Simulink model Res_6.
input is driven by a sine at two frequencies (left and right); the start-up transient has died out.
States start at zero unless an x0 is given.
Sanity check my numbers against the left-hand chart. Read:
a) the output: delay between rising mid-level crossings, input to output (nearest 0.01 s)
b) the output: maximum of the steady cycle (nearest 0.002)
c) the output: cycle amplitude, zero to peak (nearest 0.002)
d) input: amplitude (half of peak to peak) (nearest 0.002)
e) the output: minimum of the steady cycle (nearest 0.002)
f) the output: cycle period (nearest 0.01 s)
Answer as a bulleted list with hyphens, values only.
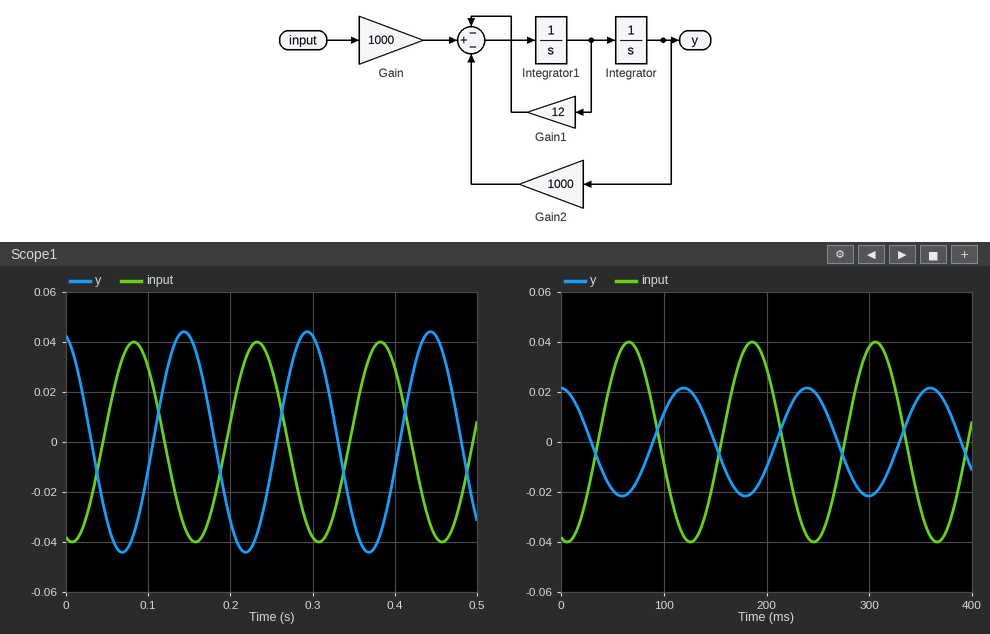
- 0.06 s
- 0.044
- 0.044
- 0.040
- -0.044
- 0.15 s
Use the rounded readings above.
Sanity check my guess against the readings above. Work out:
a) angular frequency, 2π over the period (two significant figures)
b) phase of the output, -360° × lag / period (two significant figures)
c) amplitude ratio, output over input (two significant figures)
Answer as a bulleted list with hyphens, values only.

- 42 rad/s
- -140°
- 1.1
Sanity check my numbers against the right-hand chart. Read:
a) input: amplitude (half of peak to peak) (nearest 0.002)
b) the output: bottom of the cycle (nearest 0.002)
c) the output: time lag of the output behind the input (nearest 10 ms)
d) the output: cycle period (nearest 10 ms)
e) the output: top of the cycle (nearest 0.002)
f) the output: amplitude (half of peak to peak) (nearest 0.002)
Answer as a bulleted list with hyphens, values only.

- 0.040
- -0.022
- 50 ms
- 120 ms
- 0.022
- 0.022
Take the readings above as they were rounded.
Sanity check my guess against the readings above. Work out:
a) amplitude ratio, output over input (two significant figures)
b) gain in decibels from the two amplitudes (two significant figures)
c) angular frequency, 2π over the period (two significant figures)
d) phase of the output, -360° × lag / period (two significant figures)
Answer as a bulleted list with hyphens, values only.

- 0.55
- -5.2 dB
- 0.052 rad/ms
- -150°
